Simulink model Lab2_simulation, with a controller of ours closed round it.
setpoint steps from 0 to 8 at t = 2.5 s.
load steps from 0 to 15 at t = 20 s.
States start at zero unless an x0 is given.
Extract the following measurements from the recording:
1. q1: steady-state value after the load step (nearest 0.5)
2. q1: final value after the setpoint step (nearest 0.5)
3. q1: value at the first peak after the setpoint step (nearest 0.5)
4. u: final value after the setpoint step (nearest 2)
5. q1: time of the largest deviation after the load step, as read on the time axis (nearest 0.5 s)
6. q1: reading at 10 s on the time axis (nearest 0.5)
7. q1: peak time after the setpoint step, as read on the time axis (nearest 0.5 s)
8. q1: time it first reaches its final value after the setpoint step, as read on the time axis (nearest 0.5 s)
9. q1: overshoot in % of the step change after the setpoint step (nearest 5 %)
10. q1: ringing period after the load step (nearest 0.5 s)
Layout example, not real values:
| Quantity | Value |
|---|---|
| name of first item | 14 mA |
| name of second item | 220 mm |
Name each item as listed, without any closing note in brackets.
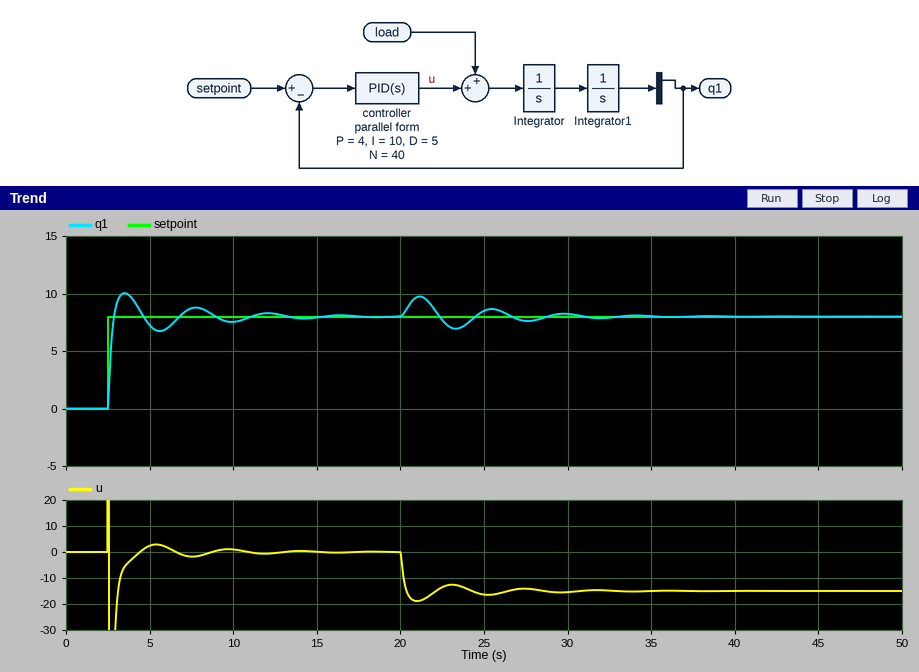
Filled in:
| Quantity | Value |
|---|---|
| q1: steady-state value after the load step | 8.0 |
| q1: final value after the setpoint step | 8.0 |
| q1: value at the first peak after the setpoint step | 10.0 |
| u: final value after the setpoint step | 0 |
| q1: time of the largest deviation after the load step, as read on the time axis | 21.0 s |
| q1: reading at 10 s on the time axis | 7.5 |
| q1: peak time after the setpoint step, as read on the time axis | 3.5 s |
| q1: time it first reaches its final value after the setpoint step, as read on the time axis | 3.0 s |
| q1: overshoot in % of the step change after the setpoint step | 25 % |
| q1: ringing period after the load step | 4.5 s |
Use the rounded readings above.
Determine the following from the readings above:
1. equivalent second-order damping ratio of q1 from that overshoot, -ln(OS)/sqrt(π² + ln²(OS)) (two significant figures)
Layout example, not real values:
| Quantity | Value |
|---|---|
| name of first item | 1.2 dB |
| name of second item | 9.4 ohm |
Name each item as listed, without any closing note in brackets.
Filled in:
| Quantity | Value |
|---|---|
| equivalent second-order damping ratio of q1 from that overshoot, -ln(OS)/sqrt(π² + ln²(OS)) | 0.40 |
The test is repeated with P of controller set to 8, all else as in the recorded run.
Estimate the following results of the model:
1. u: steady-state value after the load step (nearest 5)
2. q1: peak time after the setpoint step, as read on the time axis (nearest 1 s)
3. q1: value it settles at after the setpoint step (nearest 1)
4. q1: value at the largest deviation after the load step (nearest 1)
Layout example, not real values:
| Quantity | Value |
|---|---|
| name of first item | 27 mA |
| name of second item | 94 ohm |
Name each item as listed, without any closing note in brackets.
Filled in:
| Quantity | Value |
|---|---|
| u: steady-state value after the load step | -15 |
| q1: peak time after the setpoint step, as read on the time axis | 3 s |
| q1: value it settles at after the setpoint step | 8 |
| q1: value at the largest deviation after the load step | 9 |
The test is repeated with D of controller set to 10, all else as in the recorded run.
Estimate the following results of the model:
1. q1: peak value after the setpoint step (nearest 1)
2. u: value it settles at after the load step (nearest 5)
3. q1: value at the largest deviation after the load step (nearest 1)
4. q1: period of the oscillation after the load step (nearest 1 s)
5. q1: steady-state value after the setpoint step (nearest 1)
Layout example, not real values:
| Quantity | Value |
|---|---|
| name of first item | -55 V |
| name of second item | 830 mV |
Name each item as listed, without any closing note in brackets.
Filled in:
| Quantity | Value |
|---|---|
| q1: peak value after the setpoint step | 9 |
| u: value it settles at after the load step | -15 |
| q1: value at the largest deviation after the load step | 9 |
| q1: period of the oscillation after the load step | 6 s |
| q1: steady-state value after the setpoint step | 8 |
